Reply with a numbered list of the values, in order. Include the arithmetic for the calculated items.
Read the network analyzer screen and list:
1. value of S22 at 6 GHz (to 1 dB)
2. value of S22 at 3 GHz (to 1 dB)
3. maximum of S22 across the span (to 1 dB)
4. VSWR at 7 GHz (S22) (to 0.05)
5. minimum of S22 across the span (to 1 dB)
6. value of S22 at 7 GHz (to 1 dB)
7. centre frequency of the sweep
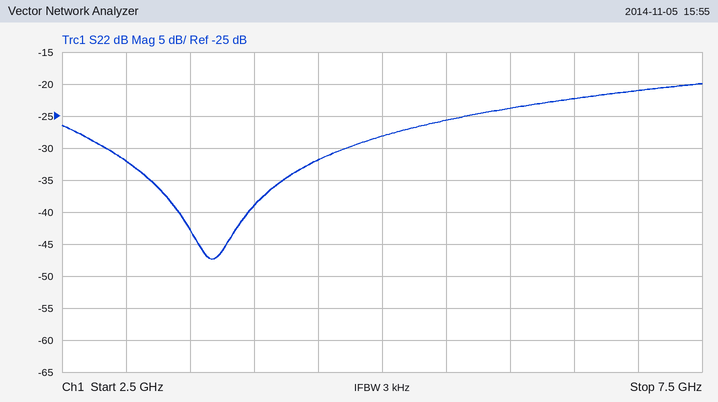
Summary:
1. -24 dB
2. -32 dB
3. -20 dB
4. |Γ| = 10^(-21/20) = 0.0891; VSWR = (1 + 0.0891)/(1 − 0.0891) ≈ 1.20
5. -47 dB
6. -21 dB
7. 5 GHz
